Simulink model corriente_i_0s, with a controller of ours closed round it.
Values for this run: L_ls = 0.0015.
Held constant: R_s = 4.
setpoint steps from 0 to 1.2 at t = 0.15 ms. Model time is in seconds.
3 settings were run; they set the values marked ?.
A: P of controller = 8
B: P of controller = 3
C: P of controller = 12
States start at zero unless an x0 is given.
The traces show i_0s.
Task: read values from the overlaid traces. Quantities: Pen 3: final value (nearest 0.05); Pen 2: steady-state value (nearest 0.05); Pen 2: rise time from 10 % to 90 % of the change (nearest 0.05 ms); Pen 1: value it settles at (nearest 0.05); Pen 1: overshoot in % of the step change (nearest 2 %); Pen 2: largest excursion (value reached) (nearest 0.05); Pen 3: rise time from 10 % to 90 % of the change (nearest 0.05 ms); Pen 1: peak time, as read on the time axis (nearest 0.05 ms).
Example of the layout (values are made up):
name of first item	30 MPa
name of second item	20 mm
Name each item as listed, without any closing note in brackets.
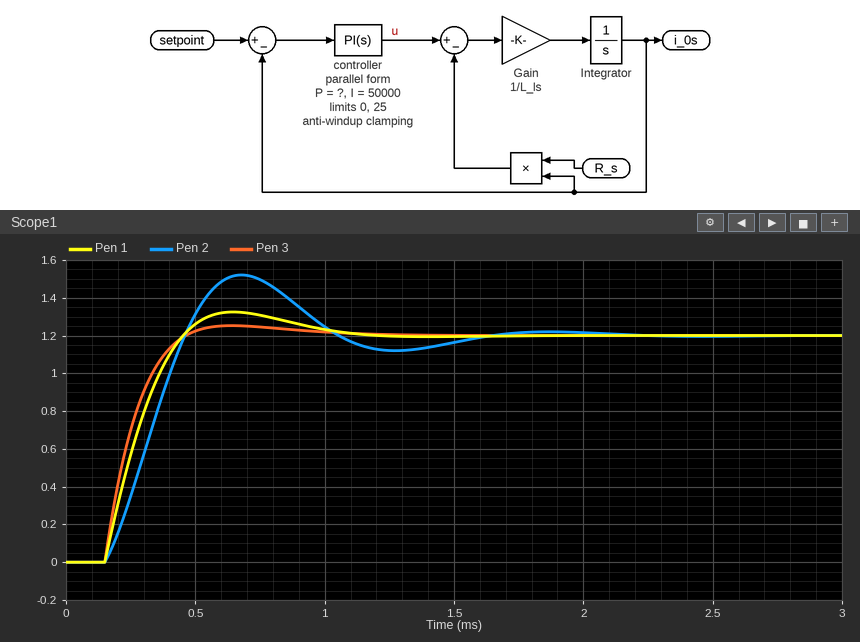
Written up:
Pen 3: final value	1.20
Pen 2: steady-state value	1.20
Pen 2: rise time from 10 % to 90 % of the change	0.25 ms
Pen 1: value it settles at	1.20
Pen 1: overshoot in % of the step change	10 %
Pen 2: largest excursion (value reached)	1.50
Pen 3: rise time from 10 % to 90 % of the change	0.20 ms
Pen 1: peak time, as read on the time axis	0.65 ms
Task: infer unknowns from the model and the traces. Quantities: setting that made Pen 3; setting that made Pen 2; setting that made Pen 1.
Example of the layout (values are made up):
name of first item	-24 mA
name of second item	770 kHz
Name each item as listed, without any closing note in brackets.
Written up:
setting that made Pen 3	C
setting that made Pen 2	B
setting that made Pen 1	A
